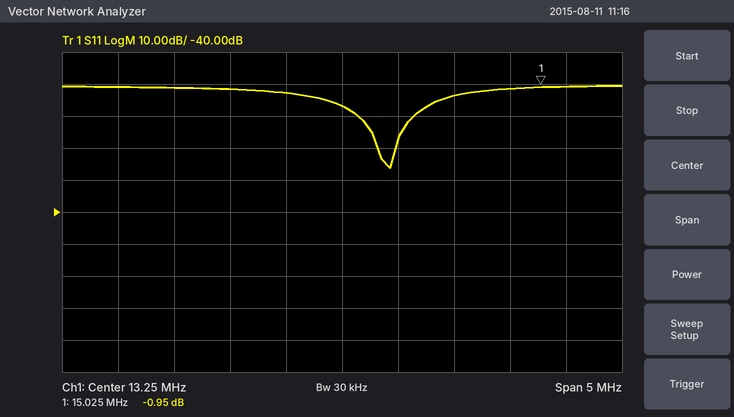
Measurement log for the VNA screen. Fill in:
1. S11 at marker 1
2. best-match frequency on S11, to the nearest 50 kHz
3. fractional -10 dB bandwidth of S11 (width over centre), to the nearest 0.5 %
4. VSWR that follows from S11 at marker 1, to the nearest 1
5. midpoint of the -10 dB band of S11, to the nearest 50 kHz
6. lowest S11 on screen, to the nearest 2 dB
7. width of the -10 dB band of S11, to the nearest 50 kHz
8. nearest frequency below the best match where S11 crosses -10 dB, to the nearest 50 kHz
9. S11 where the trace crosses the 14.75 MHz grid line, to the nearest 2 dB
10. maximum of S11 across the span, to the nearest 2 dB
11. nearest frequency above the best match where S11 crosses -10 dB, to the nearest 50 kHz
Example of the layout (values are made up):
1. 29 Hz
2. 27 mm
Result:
1. -0.95 dB
2. 13.70 MHz
3. 3.5 %
4. 18
5. 13.65 MHz
6. -26 dB
7. 500 kHz
8. 13.40 MHz
9. -2 dB
10. 0 dB
11. 13.90 MHz
